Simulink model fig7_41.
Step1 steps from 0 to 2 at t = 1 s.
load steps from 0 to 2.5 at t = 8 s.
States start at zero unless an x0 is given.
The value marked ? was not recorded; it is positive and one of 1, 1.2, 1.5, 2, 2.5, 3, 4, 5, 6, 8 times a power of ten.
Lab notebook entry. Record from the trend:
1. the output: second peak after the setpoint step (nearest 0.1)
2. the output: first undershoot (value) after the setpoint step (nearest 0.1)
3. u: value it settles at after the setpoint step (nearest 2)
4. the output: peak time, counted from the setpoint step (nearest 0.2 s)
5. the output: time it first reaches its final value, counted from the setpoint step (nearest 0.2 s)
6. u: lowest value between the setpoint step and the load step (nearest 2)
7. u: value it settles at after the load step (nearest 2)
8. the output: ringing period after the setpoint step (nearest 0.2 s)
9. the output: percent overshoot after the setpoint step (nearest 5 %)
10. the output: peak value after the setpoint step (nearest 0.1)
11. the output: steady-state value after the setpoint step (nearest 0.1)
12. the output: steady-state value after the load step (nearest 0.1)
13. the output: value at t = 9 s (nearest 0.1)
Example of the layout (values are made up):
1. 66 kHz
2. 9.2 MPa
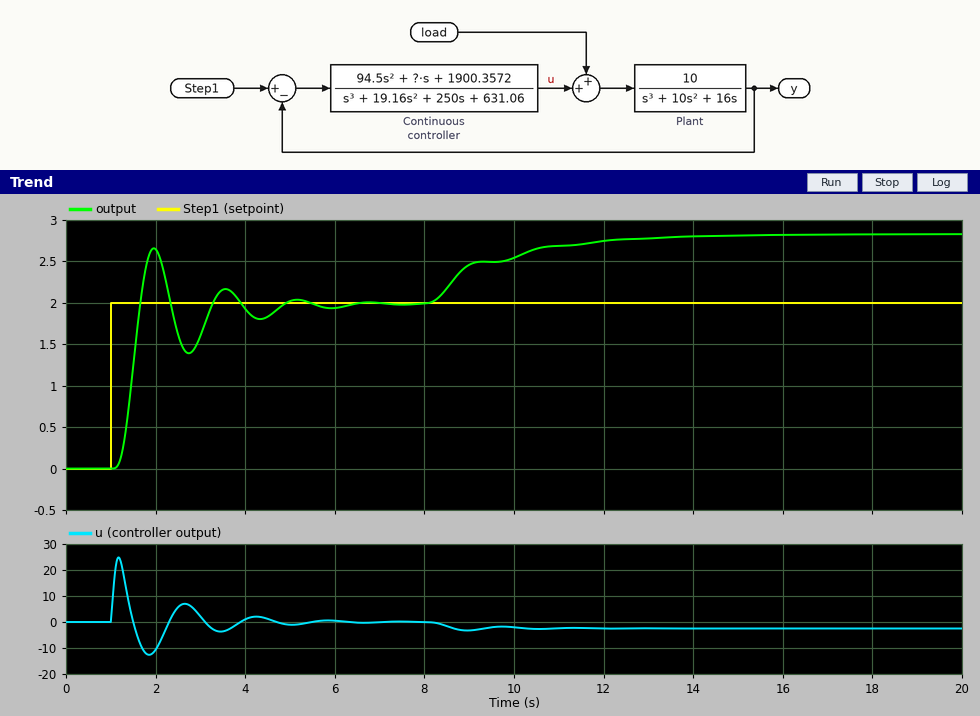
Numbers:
1. 2.2
2. 1.4
3. 0
4. 1.0 s
5. 0.6 s
6. -12
7. -2
8. 1.6 s
9. 35 %
10. 2.7
11. 2.0
12. 2.8
13. 2.5
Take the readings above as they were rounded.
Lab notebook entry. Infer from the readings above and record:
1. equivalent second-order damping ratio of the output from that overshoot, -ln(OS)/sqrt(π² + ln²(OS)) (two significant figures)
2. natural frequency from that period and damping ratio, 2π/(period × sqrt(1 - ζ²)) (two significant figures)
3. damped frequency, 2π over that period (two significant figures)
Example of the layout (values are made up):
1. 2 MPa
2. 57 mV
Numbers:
1. 0.32
2. 4.1 rad/s
3. 3.9 rad/s
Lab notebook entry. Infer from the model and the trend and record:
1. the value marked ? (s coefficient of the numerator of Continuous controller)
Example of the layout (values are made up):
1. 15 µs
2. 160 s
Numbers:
1. 3000
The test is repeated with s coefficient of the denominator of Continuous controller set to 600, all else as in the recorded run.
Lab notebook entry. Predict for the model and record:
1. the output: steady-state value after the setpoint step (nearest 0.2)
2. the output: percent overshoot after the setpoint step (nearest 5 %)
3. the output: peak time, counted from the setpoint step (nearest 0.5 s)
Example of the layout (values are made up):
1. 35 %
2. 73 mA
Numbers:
1. 2.0
2. 25 %
3. 1.5 s
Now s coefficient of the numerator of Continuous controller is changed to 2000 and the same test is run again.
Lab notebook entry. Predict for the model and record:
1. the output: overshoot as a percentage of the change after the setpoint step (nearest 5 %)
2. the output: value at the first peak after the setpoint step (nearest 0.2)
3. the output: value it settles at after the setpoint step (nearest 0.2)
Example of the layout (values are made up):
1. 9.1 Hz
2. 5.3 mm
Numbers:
1. 20 %
2. 2.4
3. 2.0
